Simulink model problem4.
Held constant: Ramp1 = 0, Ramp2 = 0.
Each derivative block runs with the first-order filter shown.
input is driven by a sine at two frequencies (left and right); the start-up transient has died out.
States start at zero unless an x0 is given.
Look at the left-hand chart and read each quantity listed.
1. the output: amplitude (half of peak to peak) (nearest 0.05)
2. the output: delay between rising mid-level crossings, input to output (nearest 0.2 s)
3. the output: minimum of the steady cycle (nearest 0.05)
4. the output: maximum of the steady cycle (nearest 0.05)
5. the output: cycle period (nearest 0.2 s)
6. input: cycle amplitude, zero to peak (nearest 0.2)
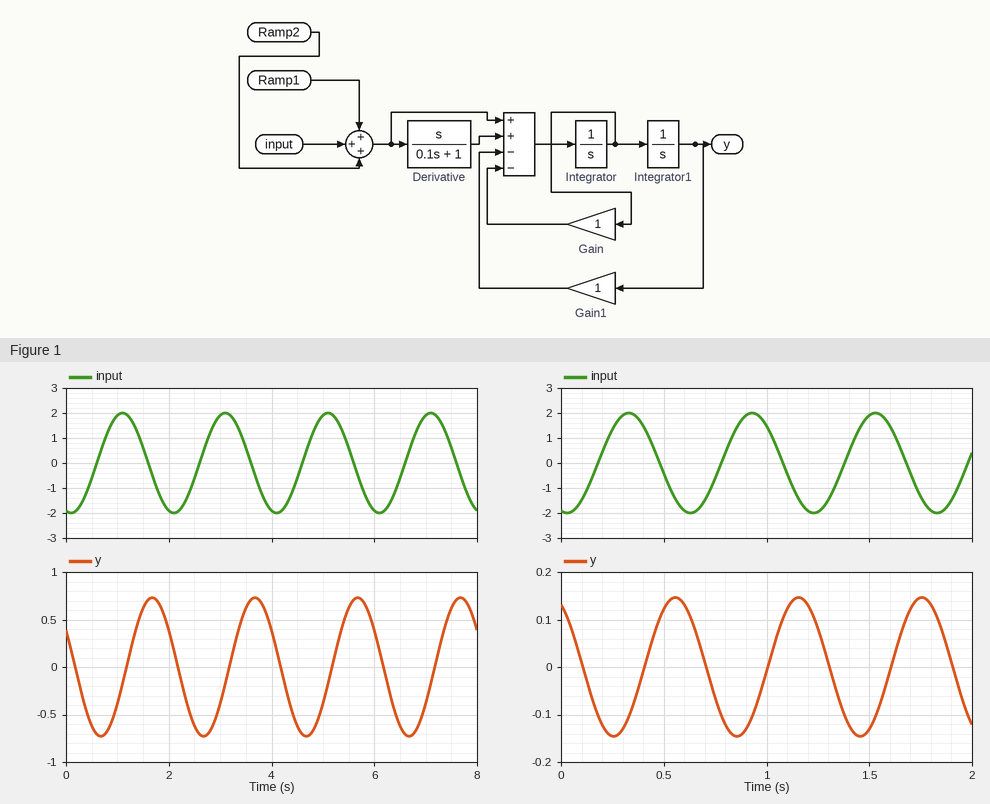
0.75
0.6 s
-0.75
0.75
2.0 s
2.0
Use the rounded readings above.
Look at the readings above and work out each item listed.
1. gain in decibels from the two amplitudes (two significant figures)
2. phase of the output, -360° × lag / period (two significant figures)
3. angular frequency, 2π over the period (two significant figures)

-8.5 dB
-110°
3.1 rad/s
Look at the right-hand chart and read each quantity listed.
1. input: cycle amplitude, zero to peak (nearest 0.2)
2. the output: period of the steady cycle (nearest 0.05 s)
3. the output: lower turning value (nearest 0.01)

2.0
0.60 s
-0.15
